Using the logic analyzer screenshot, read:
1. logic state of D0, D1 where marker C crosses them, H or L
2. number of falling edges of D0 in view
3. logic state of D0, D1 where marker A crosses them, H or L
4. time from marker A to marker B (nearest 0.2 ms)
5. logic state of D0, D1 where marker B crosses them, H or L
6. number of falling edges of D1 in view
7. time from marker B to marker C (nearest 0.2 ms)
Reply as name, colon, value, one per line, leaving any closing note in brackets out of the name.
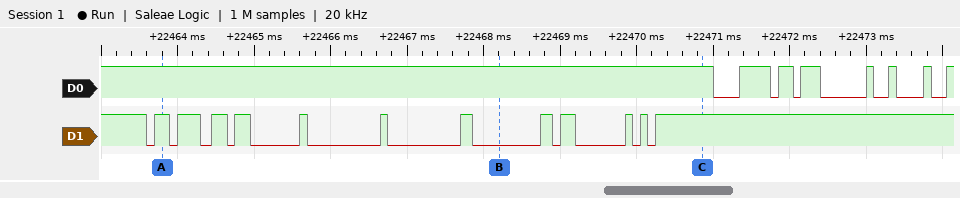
logic state of D0, D1 where marker C crosses them, H or L: D0=H, D1=H
number of falling edges of D0 in view: 7
logic state of D0, D1 where marker A crosses them, H or L: D0=H, D1=H
time from marker A to marker B: 4.4 ms
logic state of D0, D1 where marker B crosses them, H or L: D0=H, D1=L
number of falling edges of D1 in view: 12
time from marker B to marker C: 2.6 ms
